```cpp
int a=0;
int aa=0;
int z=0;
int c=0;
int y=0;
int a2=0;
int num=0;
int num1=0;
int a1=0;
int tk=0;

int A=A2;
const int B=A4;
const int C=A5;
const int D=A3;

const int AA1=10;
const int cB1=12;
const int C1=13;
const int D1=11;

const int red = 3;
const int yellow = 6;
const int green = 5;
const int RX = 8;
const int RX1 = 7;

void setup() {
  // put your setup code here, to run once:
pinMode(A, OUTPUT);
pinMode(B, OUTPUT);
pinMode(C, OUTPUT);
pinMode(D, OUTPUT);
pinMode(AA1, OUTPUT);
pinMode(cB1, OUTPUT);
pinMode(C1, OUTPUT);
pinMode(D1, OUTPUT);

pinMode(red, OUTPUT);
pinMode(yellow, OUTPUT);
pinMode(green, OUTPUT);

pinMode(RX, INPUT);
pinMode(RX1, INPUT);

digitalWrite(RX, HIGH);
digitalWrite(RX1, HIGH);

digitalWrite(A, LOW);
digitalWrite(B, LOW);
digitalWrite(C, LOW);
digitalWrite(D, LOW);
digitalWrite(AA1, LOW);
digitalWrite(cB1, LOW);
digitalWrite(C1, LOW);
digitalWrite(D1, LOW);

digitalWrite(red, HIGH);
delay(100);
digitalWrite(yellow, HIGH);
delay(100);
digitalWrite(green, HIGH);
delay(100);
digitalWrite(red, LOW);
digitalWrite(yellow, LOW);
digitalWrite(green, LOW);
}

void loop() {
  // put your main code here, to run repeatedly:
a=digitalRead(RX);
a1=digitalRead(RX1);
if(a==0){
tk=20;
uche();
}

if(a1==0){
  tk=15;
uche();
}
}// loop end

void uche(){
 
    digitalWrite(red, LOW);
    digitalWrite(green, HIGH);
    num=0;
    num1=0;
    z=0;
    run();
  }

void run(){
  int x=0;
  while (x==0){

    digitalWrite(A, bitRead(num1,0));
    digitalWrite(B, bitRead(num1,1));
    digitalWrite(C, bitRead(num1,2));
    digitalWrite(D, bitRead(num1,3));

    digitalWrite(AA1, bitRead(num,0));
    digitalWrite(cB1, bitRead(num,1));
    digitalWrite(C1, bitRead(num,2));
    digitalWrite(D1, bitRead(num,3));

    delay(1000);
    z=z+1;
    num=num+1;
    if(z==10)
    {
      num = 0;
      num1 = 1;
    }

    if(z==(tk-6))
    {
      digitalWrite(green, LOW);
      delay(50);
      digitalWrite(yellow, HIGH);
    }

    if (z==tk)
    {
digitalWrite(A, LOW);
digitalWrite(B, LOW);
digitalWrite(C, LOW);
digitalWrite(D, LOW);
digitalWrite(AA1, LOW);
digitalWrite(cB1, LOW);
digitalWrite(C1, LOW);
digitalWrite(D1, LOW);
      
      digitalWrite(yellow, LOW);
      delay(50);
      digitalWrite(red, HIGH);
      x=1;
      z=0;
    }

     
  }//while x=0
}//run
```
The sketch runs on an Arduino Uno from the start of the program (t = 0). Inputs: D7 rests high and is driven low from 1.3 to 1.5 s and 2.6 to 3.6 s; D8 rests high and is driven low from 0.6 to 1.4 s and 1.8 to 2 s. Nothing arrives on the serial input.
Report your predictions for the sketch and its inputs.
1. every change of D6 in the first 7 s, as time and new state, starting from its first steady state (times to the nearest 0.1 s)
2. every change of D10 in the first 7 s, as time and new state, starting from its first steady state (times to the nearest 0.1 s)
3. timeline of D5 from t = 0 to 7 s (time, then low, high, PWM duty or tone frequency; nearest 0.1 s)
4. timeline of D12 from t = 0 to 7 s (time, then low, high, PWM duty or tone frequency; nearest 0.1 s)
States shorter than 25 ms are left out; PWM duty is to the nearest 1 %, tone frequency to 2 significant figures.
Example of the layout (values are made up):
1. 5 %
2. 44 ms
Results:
1. 0 s low; 0.1 s high; 0.3 s low
2. 0 s low; 1.6 s high; 2.6 s low; 3.6 s high; 4.6 s low; 5.6 s high; 6.6 s low
3. 0 s low; 0.2 s high; 0.3 s low; 0.6 s high
4. 0 s low; 2.6 s high; 4.6 s low; 6.6 s high
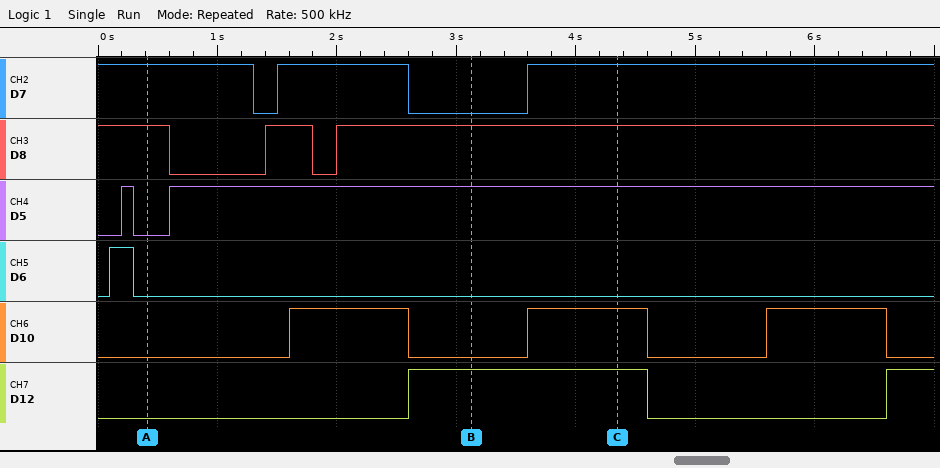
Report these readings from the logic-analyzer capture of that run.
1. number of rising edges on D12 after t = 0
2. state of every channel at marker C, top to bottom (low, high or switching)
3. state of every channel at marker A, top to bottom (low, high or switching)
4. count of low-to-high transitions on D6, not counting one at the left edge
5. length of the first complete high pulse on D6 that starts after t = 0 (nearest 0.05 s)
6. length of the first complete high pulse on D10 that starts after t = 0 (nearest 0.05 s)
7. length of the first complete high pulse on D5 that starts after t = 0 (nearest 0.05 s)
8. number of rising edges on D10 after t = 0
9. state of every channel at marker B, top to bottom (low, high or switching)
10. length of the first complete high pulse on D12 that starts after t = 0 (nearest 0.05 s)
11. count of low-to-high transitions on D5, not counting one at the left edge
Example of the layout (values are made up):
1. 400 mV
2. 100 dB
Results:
1. 2
2. D7 high, D8 high, D5 high, D6 low, D10 high, D12 high
3. D7 high, D8 high, D5 low, D6 low, D10 low, D12 low
4. 1
5. 0.20 s
6. 1.00 s
7. 0.10 s
8. 3
9. D7 low, D8 high, D5 high, D6 low, D10 low, D12 high
10. 2.00 s
11. 2
